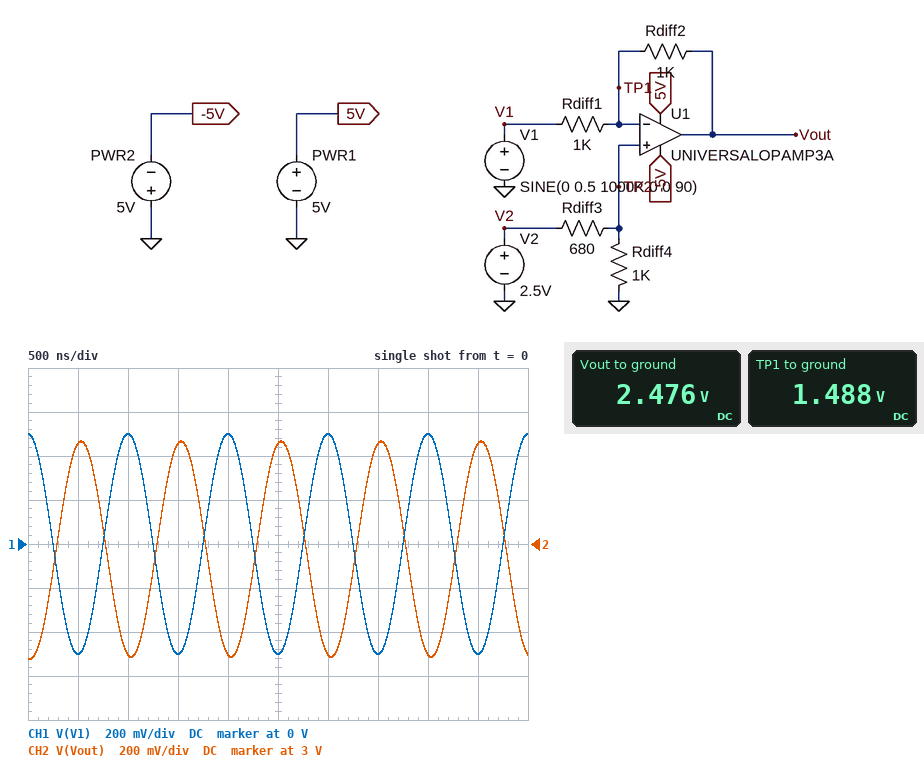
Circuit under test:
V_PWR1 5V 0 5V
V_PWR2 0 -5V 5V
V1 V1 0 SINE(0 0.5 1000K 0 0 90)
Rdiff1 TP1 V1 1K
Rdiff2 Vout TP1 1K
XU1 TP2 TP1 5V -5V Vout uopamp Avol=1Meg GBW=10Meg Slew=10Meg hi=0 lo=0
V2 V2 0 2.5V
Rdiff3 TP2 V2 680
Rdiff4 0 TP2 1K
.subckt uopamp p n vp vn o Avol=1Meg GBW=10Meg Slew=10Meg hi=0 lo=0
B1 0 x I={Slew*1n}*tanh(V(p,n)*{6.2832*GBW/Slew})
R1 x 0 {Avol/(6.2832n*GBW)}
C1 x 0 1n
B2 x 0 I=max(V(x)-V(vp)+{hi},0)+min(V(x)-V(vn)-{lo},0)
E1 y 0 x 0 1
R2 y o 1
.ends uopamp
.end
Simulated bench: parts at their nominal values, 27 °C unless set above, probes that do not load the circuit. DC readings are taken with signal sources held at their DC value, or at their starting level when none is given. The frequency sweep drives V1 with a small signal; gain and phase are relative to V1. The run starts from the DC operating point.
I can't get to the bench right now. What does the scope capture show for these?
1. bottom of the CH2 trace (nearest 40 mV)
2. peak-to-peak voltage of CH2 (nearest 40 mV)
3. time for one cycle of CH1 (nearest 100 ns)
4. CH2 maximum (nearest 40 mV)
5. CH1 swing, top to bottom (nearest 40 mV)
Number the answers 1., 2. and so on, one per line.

1. 2.48 V
2. 1.00 V
3. 1.0 µs
4. 3.48 V
5. 1.00 V
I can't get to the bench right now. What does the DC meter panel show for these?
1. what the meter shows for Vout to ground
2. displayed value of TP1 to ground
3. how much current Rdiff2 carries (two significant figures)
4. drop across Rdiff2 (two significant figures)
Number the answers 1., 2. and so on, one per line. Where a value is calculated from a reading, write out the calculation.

1. 2.476 V
2. 1.488 V
3. (2.476 V - 1.488 V) / 1 kΩ = 990 µA
4. 2.476 V - 1.488 V = 990 mV
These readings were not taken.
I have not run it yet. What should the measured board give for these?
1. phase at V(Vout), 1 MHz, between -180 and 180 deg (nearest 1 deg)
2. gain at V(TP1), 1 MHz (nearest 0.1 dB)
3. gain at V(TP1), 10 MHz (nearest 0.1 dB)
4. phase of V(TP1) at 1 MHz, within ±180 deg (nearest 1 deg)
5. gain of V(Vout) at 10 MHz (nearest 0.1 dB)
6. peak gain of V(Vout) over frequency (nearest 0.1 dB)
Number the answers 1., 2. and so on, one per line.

1. 169 deg
2. -20.2 dB
3. -7.0 dB
4. 79 deg
5. -7.0 dB
6. 0 dB
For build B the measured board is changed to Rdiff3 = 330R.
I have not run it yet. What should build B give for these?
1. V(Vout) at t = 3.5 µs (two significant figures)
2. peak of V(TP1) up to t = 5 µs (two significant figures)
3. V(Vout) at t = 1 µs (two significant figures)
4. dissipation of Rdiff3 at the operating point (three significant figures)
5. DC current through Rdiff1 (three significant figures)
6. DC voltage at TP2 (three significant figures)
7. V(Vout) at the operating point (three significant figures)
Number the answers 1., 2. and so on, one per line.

1. 4.2 V
2. 1.9 V
3. 3.3 V
4. 1.17 mW
5. 1.38 mA
6. 1.88 V
7. 3.26 V
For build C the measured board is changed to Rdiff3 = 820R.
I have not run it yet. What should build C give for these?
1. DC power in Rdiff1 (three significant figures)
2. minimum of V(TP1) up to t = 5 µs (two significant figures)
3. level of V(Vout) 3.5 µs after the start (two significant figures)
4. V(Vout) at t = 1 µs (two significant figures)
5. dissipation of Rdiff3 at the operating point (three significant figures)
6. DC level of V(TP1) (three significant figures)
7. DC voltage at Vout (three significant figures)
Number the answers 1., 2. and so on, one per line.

1. 763 µW
2. 1.3 V
3. 3.2 V
4. 2.3 V
5. 1.55 mW
6. 1.37 V
7. 2.25 V
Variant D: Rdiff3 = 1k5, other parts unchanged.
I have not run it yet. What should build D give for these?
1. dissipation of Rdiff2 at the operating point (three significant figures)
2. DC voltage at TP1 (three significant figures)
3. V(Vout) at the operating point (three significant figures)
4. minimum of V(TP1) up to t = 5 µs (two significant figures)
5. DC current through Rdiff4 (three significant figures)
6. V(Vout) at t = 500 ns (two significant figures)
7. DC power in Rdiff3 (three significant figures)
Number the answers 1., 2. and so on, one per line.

1. 250 µW
2. 1.00 V
3. 1.50 V
4. 950 mV
5. 1.00 mA
6. 2.5 V
7. 1.50 mW
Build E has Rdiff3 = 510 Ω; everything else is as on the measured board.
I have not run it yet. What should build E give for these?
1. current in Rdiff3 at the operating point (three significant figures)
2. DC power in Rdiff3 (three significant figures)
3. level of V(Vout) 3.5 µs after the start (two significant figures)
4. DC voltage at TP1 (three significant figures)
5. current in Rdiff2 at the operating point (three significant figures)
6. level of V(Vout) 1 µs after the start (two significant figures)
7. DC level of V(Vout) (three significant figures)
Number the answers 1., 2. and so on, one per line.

1. 1.66 mA
2. 1.40 mW
3. 3.8 V
4. 1.66 V
5. 1.16 mA
6. 2.8 V
7. 2.81 V
